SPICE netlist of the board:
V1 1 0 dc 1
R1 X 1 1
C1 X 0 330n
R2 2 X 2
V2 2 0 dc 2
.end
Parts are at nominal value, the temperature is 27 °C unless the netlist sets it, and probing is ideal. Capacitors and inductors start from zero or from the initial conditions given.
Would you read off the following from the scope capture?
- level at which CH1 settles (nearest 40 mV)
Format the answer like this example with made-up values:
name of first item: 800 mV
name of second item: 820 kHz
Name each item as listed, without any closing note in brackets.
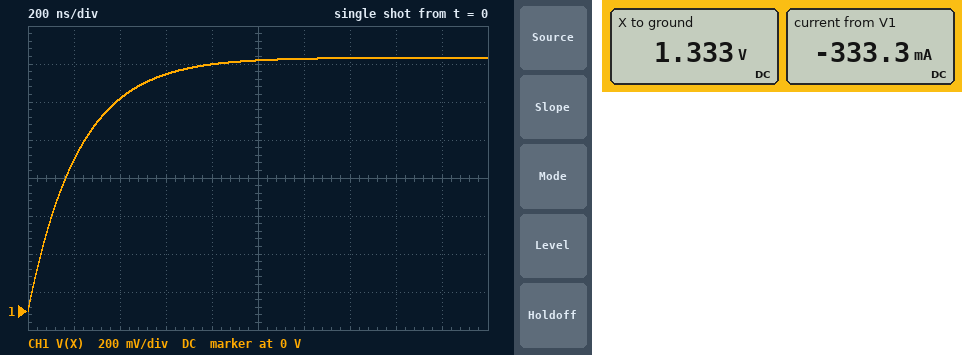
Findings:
level at which CH1 settles: 1.32 V
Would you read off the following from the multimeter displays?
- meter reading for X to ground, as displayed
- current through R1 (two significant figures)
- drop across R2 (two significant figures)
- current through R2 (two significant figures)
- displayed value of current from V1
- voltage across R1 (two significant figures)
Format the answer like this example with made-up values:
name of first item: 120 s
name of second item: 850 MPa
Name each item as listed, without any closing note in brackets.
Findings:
meter reading for X to ground, as displayed: 1.333 V
current through R1: 330 mA
drop across R2: 670 mV
current through R2: 330 mA
displayed value of current from V1: -333.3 mA
voltage across R1: 330 mV
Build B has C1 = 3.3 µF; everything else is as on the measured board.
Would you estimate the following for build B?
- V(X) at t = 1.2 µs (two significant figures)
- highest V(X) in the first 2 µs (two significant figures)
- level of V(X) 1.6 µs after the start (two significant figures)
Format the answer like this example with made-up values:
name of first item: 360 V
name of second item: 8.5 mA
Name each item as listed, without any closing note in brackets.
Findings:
V(X) at t = 1.2 µs: 560 mV
highest V(X) in the first 2 µs: 800 mV
level of V(X) 1.6 µs after the start: 690 mV
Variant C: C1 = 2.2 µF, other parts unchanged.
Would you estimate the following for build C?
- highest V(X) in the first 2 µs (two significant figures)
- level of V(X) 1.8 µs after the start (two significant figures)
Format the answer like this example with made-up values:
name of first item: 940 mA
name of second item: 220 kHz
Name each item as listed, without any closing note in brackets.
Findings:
highest V(X) in the first 2 µs: 990 mV
level of V(X) 1.8 µs after the start: 940 mV
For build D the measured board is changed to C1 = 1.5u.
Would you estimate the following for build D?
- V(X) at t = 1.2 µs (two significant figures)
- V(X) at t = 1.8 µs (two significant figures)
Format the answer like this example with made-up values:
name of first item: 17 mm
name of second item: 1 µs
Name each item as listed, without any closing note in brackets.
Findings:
V(X) at t = 1.2 µs: 930 mV
V(X) at t = 1.8 µs: 1.1 V
